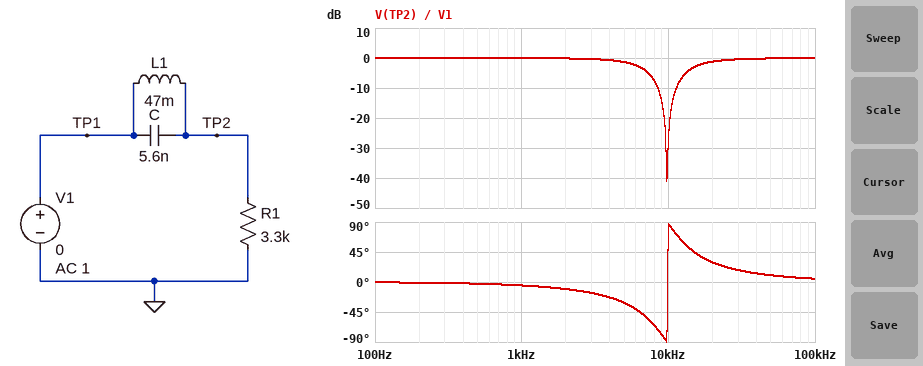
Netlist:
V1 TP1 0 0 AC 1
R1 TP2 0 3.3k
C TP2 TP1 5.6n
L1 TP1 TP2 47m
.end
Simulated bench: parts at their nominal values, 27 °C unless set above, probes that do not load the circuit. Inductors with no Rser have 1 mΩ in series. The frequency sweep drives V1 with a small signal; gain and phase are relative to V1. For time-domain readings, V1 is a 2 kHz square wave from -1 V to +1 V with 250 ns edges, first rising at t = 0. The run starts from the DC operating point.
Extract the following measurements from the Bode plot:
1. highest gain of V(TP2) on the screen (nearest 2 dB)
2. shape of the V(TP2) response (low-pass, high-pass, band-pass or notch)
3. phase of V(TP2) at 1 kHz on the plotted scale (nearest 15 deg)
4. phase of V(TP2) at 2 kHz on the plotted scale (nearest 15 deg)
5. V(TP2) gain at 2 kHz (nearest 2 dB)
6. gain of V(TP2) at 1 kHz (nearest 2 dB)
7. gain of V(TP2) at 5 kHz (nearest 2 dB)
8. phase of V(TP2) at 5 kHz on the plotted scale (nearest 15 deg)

0 dB
notch
0 deg
-15 deg
0 dB
0 dB
-2 dB
-30 deg
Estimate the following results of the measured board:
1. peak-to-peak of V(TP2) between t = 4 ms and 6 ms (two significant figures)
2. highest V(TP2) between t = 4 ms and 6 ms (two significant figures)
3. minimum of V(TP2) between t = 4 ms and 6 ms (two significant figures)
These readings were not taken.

2.4 V
1.2 V
-1.2 V
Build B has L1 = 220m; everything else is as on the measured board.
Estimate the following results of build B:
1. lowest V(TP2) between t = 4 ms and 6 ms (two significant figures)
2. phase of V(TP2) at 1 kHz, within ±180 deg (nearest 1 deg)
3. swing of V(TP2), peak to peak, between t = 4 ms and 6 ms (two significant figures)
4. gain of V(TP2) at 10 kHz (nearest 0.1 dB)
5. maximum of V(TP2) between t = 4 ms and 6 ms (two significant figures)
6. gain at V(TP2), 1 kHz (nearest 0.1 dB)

-1.0 V
-24 deg
2.0 V
-3.4 dB
1.0 V
-0.8 dB
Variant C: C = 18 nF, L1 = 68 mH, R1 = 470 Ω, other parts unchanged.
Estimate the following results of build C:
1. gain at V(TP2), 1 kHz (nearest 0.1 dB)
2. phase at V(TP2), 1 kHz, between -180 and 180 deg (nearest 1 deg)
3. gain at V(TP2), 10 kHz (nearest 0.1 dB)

-2.8 dB
-44 deg
-8.2 dB
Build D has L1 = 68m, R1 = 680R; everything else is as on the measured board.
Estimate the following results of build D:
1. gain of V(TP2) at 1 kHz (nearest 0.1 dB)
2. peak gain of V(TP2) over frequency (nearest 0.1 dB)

-1.5 dB
0 dB
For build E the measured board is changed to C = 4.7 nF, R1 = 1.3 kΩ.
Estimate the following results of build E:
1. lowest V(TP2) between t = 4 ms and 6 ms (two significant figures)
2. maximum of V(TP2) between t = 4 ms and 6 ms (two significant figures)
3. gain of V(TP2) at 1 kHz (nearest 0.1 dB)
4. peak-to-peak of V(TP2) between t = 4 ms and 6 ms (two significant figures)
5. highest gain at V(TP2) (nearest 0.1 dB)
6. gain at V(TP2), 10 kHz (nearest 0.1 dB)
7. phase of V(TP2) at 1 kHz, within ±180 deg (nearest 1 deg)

-1.0 V
1.0 V
-0.2 dB
2.0 V
0 dB
-25.0 dB
-13 deg
